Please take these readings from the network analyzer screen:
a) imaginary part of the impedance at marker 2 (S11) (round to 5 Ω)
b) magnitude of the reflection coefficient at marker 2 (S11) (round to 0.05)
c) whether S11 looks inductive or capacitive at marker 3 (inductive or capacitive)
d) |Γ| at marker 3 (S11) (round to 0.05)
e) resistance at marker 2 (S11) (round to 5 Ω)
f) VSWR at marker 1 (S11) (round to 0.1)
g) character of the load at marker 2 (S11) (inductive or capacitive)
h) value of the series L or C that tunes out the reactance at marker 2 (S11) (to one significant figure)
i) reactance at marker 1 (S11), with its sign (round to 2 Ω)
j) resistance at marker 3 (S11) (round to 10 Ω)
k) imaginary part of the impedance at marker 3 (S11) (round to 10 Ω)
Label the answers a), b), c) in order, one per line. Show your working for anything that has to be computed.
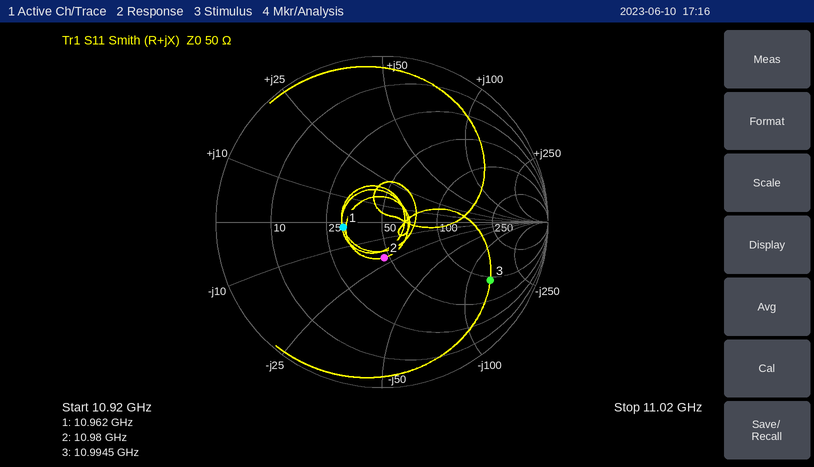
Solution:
a) -20 Ω
b) 0.20
c) capacitive
d) 0.75
e) 45 Ω
f) 1.6
g) capacitive
h) L = 20 Ω/(2π × 10.98 GHz) ≈ 290 pH, so 300 pH to one significant figure
i) -2 Ω
j) 90 Ω
k) -140 Ω
